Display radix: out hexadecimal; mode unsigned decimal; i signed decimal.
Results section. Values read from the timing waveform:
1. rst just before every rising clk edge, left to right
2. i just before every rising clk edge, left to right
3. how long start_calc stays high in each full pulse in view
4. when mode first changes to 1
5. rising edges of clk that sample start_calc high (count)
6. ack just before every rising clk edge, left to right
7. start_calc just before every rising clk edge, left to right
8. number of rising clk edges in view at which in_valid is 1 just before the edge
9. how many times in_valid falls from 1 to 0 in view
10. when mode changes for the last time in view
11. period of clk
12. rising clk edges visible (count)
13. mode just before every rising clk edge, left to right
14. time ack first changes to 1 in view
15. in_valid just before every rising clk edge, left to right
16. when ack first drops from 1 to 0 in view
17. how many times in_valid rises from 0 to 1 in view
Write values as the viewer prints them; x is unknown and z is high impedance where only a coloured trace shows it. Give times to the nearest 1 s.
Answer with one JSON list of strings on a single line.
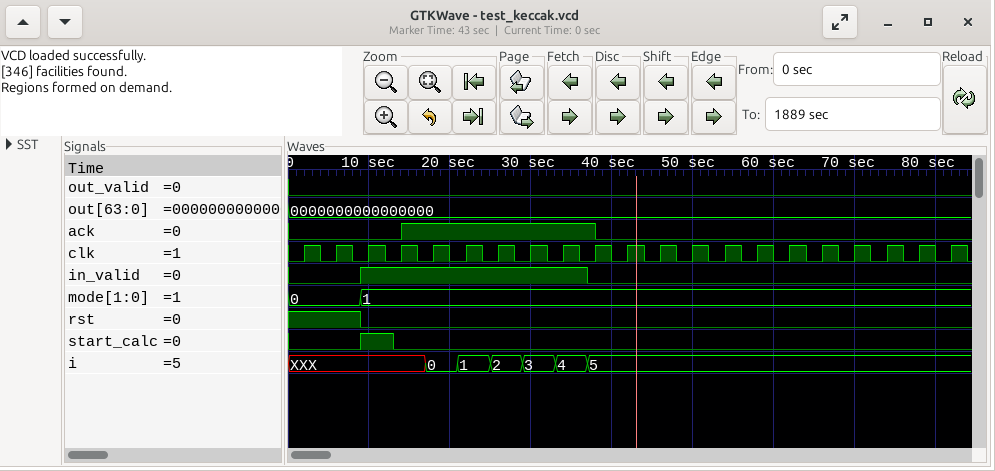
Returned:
["1 1 0 0 0 0 0 0 0 0 0 0 0 0 0 0 0 0 0 0 0", "XXX, XXX, XXX, XXX, 0, 1, 2, 3, 4, 5, 5, 5, 5, 5, 5, 5, 5, 5, 5, 5, 5", "4 s", "9 s", "1", "0 0 0 0 1 1 1 1 1 1 0 0 0 0 0 0 0 0 0 0 0", "0 0 1 0 0 0 0 0 0 0 0 0 0 0 0 0 0 0 0 0 0", "7", "1", "9 s", "4 s", "21", "0, 0, 1, 1, 1, 1, 1, 1, 1, 1, 1, 1, 1, 1, 1, 1, 1, 1, 1, 1, 1", "14 s", "0 0 1 1 1 1 1 1 1 0 0 0 0 0 0 0 0 0 0 0 0", "38 s", "1"]
